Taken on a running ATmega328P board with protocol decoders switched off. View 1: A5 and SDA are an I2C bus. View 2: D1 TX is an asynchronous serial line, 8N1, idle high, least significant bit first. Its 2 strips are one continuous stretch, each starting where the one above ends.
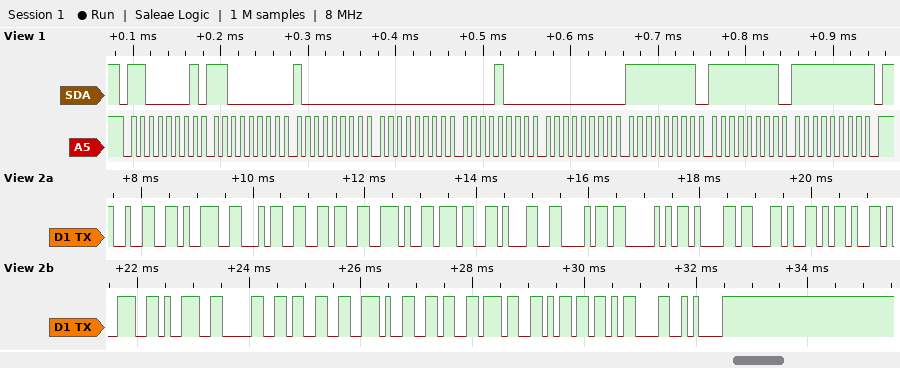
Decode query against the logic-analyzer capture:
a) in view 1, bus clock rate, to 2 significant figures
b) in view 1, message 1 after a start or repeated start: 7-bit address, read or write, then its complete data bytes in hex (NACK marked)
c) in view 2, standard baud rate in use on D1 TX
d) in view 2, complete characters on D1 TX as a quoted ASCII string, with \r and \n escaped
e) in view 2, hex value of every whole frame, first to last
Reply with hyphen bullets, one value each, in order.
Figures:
- 100 kHz
- 0x60 read: C0 80 00 08 00 FF FF FF NACK
- 9600 baud
- "2946.71hPa,-9903.67m\r\n"
- 32 39 34 36 2E 37 31 68 50 61 2C 2D 39 39 30 33 2E 36 37 6D 0D 0A
